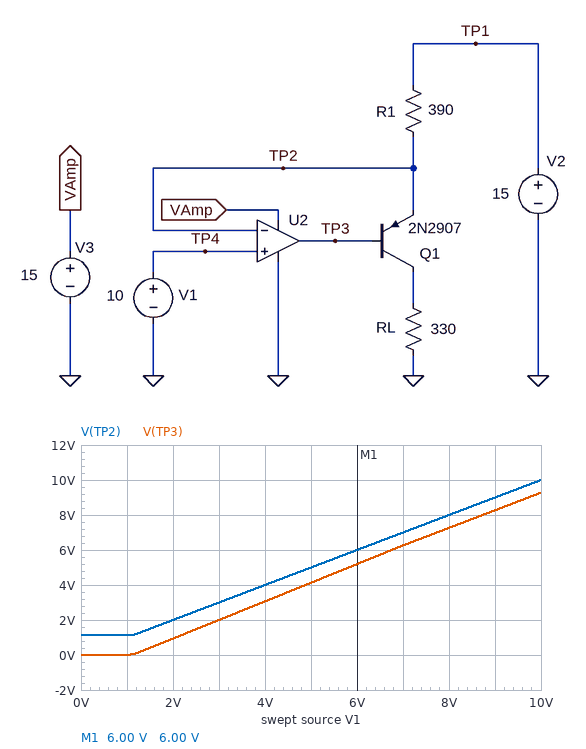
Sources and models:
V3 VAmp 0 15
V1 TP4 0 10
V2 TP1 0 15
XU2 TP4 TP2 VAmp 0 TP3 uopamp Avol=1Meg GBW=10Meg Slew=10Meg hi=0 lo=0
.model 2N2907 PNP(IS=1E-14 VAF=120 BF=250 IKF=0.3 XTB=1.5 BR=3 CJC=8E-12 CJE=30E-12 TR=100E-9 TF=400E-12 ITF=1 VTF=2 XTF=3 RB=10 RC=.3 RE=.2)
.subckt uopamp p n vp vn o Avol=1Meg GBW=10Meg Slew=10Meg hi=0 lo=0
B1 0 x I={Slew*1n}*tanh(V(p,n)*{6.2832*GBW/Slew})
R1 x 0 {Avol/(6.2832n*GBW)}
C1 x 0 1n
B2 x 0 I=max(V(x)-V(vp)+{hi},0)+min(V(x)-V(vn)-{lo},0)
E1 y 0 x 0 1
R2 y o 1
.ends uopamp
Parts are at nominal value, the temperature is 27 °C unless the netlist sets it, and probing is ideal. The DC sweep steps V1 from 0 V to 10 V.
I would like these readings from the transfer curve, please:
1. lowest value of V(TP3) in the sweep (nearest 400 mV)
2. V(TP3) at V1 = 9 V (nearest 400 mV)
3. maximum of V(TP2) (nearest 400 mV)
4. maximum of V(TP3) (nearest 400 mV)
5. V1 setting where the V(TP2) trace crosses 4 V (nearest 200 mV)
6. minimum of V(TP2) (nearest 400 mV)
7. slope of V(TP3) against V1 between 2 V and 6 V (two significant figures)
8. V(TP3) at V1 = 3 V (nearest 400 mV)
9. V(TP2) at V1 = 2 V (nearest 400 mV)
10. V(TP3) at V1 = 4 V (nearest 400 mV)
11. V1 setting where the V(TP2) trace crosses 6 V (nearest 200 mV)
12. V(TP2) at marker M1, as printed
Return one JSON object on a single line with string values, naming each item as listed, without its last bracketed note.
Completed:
{"lowest value of V(TP3) in the sweep": "0 V", "V(TP3) at V1 = 9 V": "8.4 V", "maximum of V(TP2)": "10.0 V", "maximum of V(TP3)": "9.2 V", "V1 setting where the V(TP2) trace crosses 4 V": "4.0 V", "minimum of V(TP2)": "1.2 V", "slope of V(TP3) against V1 between 2 V and 6 V": "1.1 V/V", "V(TP3) at V1 = 3 V": "2.0 V", "V(TP2) at V1 = 2 V": "2.0 V", "V(TP3) at V1 = 4 V": "3.2 V", "V1 setting where the V(TP2) trace crosses 6 V": "6.0 V", "V(TP2) at marker M1, as printed": "6.00 V"}
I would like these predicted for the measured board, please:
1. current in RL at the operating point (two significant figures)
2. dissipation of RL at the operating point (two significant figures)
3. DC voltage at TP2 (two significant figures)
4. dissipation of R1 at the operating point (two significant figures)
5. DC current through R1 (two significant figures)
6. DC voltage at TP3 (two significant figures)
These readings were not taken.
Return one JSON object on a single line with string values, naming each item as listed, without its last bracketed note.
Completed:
{"current in RL at the operating point": "13 mA", "dissipation of RL at the operating point": "54 mW", "DC voltage at TP2": "10 V", "dissipation of R1 at the operating point": "64 mW", "DC current through R1": "13 mA", "DC voltage at TP3": "9.3 V"}
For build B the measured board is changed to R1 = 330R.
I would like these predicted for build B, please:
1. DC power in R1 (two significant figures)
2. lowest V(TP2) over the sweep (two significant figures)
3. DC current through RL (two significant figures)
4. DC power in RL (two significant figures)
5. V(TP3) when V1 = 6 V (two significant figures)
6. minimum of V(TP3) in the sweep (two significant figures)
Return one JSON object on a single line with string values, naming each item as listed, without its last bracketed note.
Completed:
{"DC power in R1": "76 mW", "lowest V(TP2) over the sweep": "1.2 V", "DC current through RL": "15 mA", "DC power in RL": "75 mW", "V(TP3) when V1 = 6 V": "5.1 V", "minimum of V(TP3) in the sweep": "28 mV"}
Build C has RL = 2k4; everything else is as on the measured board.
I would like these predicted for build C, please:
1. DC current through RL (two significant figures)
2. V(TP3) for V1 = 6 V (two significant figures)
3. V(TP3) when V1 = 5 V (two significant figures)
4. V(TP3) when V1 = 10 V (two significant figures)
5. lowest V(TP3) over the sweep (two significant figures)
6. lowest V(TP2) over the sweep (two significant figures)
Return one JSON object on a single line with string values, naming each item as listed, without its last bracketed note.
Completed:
{"DC current through RL": "4.2 mA", "V(TP3) for V1 = 6 V": "5.0 V", "V(TP3) when V1 = 5 V": "4.0 V", "V(TP3) when V1 = 10 V": "9.2 V", "lowest V(TP3) over the sweep": "25 mV", "lowest V(TP2) over the sweep": "1.2 V"}
